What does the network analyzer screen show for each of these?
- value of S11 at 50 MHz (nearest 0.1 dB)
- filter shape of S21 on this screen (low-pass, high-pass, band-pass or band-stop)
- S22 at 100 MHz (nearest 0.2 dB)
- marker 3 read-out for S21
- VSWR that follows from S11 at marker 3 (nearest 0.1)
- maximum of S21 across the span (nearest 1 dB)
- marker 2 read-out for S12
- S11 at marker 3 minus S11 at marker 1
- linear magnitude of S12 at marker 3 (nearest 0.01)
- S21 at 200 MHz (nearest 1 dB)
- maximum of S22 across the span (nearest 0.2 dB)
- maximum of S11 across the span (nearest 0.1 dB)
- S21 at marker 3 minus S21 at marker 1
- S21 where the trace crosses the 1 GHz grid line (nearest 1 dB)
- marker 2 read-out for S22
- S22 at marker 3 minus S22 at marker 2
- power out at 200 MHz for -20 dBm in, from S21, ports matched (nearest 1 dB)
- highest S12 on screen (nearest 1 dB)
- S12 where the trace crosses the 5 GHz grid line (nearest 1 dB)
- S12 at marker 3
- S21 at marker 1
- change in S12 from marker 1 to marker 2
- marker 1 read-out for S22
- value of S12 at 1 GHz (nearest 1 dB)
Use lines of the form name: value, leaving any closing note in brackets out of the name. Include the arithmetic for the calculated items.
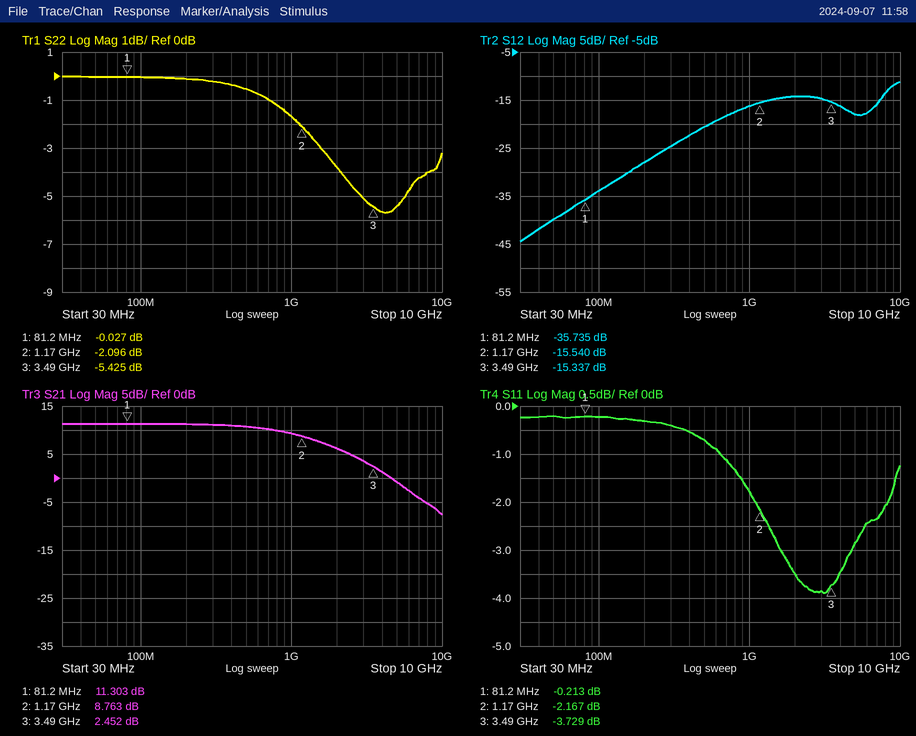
value of S11 at 50 MHz: -0.2 dB
filter shape of S21 on this screen: low-pass
S22 at 100 MHz: 0.0 dB
marker 3 read-out for S21: 2.452 dB
VSWR that follows from S11 at marker 3: (1 + 0.6510)/(1 − 0.6510) ≈ 4.7
maximum of S21 across the span: 11 dB
marker 2 read-out for S12: -15.540 dB
S11 at marker 3 minus S11 at marker 1: -3.729 − (-0.213) = -3.516 dB
linear magnitude of S12 at marker 3: 10^(-15.337/20) ≈ 0.17
S21 at 200 MHz: 11 dB
maximum of S22 across the span: 0.0 dB
maximum of S11 across the span: -0.2 dB
S21 at marker 3 minus S21 at marker 1: 2.452 − (11.303) = -8.851 dB
S21 where the trace crosses the 1 GHz grid line: 9 dB
marker 2 read-out for S22: -2.096 dB
S22 at marker 3 minus S22 at marker 2: -5.425 − (-2.096) = -3.329 dB
power out at 200 MHz for -20 dBm in, from S21, ports matched: -20 dBm + (11 dB) = -9 dBm
highest S12 on screen: -11 dB
S12 where the trace crosses the 5 GHz grid line: -18 dB
S12 at marker 3: -15.337 dB
S21 at marker 1: 11.303 dB
change in S12 from marker 1 to marker 2: -15.54 − (-35.735) = 20.195 dB
marker 1 read-out for S22: -0.027 dB
value of S12 at 1 GHz: -16 dB
